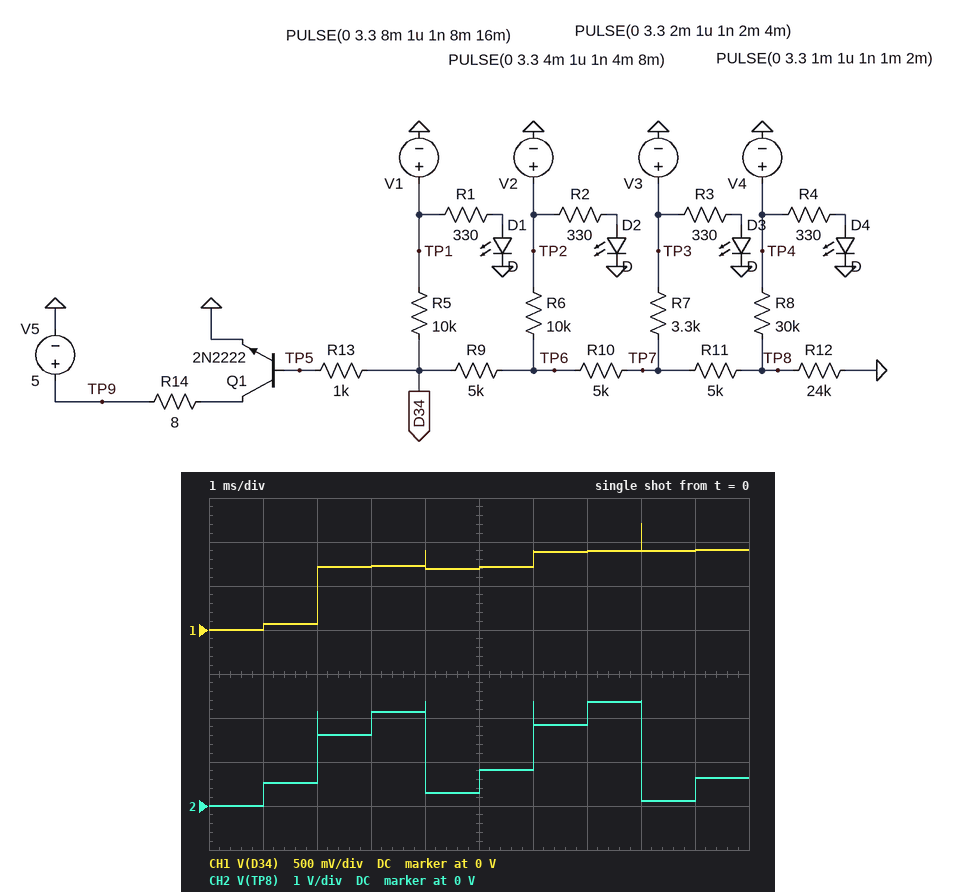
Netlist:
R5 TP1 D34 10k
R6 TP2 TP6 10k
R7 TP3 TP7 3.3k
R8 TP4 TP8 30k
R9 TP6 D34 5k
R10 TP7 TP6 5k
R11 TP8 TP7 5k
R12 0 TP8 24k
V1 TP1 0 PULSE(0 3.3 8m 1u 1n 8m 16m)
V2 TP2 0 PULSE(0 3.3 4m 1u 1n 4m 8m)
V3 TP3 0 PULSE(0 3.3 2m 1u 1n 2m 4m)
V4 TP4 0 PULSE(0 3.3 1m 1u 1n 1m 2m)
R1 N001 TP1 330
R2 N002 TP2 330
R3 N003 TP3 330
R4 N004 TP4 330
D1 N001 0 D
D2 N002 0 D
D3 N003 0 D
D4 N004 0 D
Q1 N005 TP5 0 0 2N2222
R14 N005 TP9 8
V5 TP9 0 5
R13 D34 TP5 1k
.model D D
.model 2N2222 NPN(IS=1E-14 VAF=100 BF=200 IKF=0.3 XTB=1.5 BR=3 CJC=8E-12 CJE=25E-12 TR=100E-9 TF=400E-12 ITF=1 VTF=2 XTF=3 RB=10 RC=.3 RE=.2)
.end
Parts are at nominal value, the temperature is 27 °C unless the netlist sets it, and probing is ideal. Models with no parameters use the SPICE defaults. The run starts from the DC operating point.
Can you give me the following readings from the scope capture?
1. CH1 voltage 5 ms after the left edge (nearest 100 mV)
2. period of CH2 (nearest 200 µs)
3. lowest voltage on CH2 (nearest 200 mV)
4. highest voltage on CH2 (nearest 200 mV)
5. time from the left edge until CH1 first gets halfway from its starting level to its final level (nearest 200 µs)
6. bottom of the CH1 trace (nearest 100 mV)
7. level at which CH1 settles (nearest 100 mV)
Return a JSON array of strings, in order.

["700 mV", "4.0 ms", "0 V", "2.4 V", "2.0 ms", "0 V", "900 mV"]
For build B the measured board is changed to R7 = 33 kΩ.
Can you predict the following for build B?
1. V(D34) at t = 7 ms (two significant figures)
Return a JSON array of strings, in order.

["800 mV"]
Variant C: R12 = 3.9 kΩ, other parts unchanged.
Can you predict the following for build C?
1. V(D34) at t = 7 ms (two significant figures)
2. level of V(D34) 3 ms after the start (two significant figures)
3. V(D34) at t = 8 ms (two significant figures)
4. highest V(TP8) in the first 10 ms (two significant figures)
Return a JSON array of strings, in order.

["860 mV", "670 mV", "870 mV", "1.2 V"]
